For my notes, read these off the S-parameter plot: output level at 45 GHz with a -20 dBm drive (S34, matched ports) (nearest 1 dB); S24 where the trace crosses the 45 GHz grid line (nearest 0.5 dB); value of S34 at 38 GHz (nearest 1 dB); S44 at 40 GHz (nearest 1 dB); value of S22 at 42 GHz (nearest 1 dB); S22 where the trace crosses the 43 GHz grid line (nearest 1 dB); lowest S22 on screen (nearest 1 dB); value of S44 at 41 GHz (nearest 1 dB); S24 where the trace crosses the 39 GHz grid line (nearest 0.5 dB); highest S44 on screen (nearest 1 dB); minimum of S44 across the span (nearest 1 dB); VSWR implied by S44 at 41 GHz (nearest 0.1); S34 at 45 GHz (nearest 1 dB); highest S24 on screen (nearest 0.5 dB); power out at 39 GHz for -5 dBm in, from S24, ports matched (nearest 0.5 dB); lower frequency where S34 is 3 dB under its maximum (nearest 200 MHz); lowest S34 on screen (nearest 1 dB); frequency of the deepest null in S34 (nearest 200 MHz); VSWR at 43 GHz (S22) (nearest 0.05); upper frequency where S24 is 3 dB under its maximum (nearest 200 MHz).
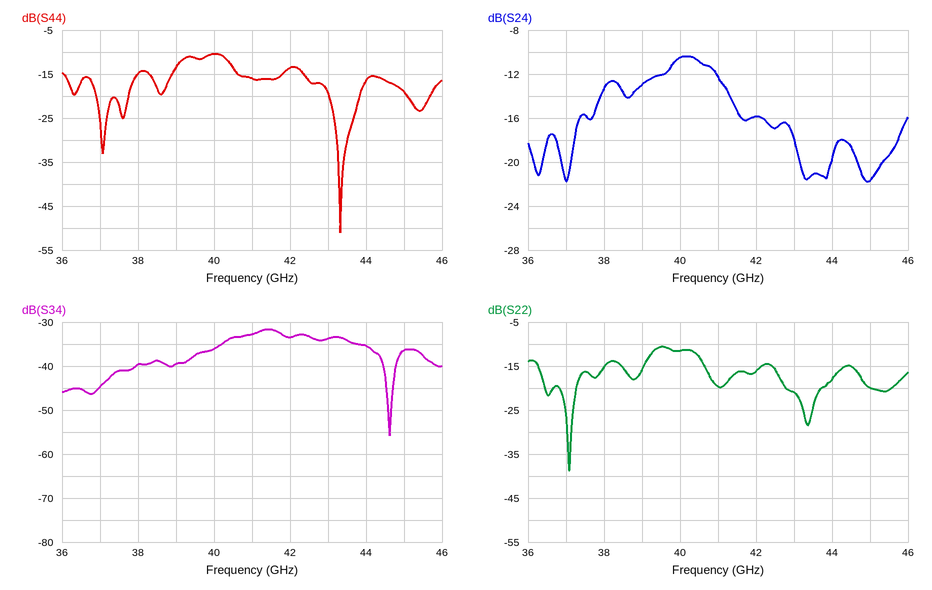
-56 dBm
-21.5 dB
-40 dB
-10 dB
-16 dB
-21 dB
-39 dB
-16 dB
-13.0 dB
-10 dB
-51 dB
1.4
-36 dB
-10.5 dB
-18.0 dBm
40.2 GHz
-56 dB
44.6 GHz
1.20
41.2 GHz
